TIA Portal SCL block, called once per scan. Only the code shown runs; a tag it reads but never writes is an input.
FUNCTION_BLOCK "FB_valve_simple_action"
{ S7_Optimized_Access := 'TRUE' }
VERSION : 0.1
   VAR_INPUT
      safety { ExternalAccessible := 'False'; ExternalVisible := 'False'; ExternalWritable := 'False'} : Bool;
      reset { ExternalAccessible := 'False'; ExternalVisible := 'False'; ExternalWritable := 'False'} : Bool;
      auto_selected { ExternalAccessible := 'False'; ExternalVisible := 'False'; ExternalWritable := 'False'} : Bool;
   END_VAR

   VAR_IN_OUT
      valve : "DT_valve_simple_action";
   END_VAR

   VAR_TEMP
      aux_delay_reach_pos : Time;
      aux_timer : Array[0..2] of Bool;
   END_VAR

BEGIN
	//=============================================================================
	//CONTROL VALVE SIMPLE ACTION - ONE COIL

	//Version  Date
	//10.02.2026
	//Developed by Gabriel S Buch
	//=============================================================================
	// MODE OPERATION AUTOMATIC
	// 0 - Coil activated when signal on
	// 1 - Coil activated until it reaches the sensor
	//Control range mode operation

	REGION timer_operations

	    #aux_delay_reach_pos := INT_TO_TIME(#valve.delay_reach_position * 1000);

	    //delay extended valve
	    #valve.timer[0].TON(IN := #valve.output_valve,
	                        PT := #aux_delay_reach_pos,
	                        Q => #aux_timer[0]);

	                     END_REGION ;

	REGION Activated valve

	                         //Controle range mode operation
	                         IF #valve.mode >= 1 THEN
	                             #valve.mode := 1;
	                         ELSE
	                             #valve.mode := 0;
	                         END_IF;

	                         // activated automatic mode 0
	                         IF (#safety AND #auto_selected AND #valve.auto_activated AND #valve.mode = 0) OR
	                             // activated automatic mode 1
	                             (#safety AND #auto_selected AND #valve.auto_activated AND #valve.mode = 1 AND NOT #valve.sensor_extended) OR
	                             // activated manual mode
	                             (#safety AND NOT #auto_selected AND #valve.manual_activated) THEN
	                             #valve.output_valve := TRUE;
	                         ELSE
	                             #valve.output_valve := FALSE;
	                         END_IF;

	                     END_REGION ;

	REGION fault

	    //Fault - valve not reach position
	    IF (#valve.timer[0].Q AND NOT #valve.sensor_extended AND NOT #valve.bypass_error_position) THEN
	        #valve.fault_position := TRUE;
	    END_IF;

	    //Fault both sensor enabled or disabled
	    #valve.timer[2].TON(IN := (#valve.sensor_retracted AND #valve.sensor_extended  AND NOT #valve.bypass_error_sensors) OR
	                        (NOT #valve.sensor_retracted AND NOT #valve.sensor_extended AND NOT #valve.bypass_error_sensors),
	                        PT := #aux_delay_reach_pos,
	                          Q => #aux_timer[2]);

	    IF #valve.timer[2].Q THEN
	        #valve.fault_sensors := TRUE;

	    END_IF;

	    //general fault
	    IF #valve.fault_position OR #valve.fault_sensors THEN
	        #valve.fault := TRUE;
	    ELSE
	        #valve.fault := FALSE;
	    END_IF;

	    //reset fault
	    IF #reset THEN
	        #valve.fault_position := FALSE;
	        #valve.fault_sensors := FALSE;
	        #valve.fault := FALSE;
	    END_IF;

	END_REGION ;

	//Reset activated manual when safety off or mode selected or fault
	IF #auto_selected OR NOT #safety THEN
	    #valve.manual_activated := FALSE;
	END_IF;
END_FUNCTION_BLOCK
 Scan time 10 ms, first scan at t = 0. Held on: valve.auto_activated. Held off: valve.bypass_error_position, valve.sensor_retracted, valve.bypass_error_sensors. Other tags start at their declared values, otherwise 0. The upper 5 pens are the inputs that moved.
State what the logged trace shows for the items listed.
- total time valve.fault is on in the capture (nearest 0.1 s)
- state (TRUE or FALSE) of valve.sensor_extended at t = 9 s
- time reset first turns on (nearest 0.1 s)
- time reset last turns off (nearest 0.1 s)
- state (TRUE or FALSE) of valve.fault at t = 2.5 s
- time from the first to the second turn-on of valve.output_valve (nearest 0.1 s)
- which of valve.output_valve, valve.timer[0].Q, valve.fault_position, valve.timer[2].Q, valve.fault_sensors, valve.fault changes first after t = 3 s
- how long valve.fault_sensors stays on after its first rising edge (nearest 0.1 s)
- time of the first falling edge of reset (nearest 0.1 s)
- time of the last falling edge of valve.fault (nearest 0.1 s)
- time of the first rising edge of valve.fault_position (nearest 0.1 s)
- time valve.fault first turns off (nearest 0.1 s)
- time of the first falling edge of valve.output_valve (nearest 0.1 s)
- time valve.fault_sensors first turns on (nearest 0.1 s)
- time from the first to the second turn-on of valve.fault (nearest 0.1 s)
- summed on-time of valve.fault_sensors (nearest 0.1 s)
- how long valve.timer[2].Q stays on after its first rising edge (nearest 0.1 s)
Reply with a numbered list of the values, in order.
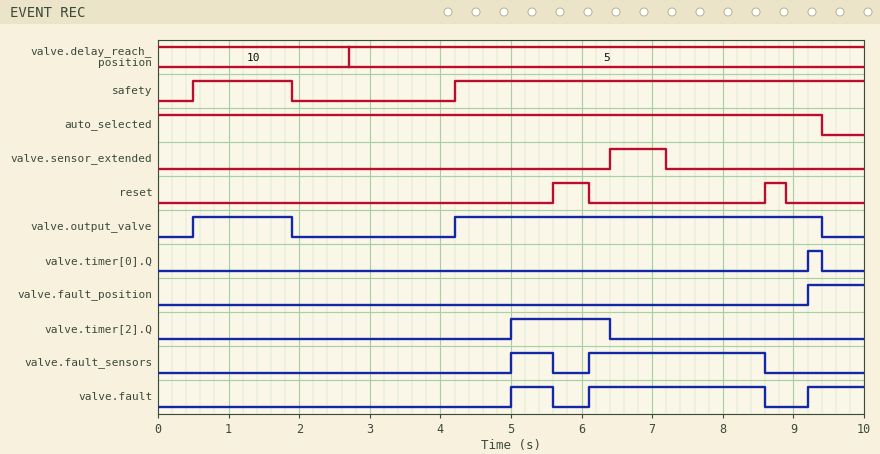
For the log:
1. 3.9 s
2. FALSE
3. 5.6 s
4. 8.9 s
5. FALSE
6. 3.7 s
7. valve.output_valve
8. 0.6 s
9. 6.1 s
10. 8.6 s
11. 9.2 s
12. 5.6 s
13. 1.9 s
14. 5.0 s
15. 1.1 s
16. 3.1 s
17. 1.4 s
